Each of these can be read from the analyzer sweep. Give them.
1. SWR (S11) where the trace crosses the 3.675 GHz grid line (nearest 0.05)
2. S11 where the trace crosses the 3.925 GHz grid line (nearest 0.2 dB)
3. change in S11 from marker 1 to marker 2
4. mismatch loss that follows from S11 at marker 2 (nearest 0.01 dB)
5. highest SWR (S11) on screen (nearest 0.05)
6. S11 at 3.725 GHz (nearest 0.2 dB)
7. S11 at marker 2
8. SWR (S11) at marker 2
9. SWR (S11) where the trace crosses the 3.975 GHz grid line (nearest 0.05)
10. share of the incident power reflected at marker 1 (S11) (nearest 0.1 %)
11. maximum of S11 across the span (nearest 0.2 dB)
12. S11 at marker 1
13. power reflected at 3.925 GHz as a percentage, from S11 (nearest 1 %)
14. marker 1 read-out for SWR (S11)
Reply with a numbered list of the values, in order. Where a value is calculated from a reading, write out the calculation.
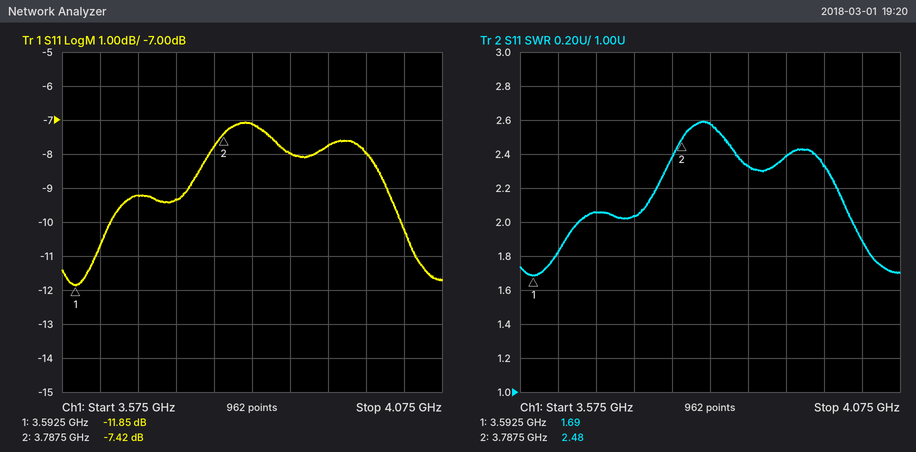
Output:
1. 2.05
2. -7.8 dB
3. -7.42 − (-11.85) = 4.43 dB
4. −10 log10(1 − 10^(-7.42/10)) ≈ 0.87 dB
5. 2.60
6. -9.4 dB
7. -7.42 dB
8. 2.48
9. 2.35
10. 10^(-11.85/10) ≈ 6.5 %
11. -7.0 dB
12. -11.85 dB
13. 10^(-7.8/10) ≈ 17 %
14. 1.69
